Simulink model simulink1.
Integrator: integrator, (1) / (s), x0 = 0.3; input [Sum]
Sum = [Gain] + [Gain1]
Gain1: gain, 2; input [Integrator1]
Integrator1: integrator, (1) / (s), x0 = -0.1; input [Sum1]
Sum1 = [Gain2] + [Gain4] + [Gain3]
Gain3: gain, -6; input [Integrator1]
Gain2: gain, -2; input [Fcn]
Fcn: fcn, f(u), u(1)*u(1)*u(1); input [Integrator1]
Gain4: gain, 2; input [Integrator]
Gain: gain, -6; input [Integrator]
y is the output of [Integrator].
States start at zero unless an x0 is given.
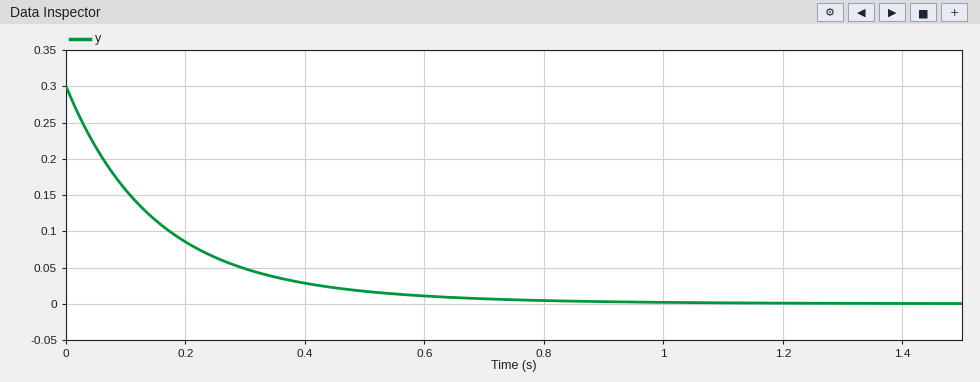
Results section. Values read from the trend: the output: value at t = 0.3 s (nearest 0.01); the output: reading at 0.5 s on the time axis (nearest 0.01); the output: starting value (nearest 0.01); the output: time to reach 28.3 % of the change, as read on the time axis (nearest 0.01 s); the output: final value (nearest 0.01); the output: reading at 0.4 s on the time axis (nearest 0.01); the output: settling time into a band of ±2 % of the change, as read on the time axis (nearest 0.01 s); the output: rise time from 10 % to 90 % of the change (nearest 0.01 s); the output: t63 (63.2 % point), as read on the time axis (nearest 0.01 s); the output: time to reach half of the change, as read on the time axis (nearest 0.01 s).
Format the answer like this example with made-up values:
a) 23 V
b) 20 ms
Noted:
a) 0.05
b) 0.02
c) 0.30
d) 0.05 s
e) 0.00
f) 0.03
g) 0.73 s
h) 0.37 s
i) 0.16 s
j) 0.11 s
